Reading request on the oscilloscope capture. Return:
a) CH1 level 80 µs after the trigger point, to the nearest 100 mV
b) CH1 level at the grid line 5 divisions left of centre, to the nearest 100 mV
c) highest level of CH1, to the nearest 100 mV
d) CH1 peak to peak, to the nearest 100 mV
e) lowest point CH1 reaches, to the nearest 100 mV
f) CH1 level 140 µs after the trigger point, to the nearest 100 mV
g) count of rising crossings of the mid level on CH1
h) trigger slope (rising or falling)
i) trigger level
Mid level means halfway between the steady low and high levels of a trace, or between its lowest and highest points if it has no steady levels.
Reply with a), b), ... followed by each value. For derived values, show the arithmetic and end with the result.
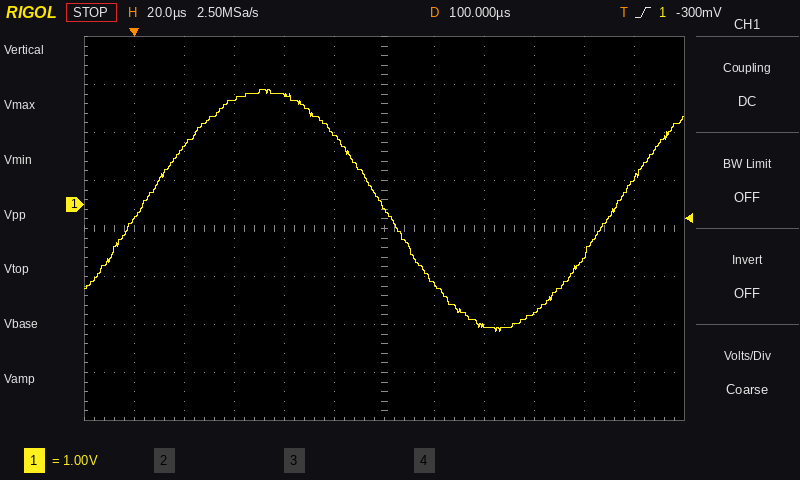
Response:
a) 1.5 V
b) -300 mV
c) 2.4 V
d) 2.4 V − (-2.6 V) = 5.0 V
e) -2.6 V
f) -2.5 V
g) 2
h) rising
i) -300 mV
